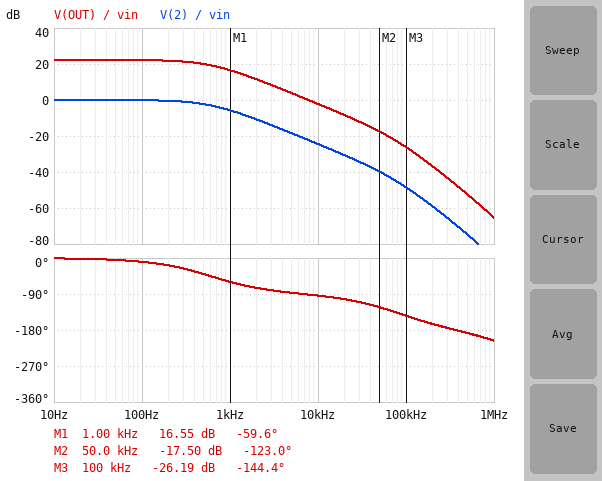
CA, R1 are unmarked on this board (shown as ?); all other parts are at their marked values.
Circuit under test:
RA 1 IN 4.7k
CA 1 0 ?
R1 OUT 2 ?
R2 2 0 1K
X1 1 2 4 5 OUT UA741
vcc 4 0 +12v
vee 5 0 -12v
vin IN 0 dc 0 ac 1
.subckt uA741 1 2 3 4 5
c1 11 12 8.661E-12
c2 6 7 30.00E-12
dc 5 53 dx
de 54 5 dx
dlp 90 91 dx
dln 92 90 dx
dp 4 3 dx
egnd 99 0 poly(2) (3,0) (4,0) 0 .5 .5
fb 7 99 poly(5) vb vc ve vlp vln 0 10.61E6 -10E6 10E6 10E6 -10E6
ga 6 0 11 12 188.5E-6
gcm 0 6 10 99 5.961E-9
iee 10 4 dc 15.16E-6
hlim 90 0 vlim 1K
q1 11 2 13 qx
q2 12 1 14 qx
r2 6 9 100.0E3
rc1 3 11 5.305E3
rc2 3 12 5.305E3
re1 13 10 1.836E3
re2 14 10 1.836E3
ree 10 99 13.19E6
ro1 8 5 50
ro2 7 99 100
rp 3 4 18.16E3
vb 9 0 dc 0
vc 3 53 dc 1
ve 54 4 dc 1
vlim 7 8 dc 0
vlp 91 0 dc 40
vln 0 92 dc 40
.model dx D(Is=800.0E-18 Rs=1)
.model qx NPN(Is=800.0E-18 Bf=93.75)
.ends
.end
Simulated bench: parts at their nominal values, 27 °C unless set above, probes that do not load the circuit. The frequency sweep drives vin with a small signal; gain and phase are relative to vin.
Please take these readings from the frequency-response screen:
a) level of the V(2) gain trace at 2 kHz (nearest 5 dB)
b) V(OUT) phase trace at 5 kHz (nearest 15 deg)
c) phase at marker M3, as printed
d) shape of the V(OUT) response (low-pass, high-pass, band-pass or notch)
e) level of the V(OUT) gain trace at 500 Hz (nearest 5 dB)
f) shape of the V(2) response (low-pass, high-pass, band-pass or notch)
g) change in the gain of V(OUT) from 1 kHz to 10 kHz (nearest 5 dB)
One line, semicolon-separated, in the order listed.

-10 dB; -90 deg; -144.4 deg; low-pass; 20 dB; low-pass; -20 dB
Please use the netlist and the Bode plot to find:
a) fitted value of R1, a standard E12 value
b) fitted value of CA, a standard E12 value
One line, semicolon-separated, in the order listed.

12 kΩ; 56 nF
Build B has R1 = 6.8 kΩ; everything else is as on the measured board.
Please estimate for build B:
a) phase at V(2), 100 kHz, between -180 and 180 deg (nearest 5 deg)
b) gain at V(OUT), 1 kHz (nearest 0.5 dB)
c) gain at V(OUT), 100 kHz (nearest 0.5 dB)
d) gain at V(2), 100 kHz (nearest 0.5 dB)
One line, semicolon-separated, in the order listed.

-130 deg; 12.0 dB; -28.5 dB; -46.0 dB
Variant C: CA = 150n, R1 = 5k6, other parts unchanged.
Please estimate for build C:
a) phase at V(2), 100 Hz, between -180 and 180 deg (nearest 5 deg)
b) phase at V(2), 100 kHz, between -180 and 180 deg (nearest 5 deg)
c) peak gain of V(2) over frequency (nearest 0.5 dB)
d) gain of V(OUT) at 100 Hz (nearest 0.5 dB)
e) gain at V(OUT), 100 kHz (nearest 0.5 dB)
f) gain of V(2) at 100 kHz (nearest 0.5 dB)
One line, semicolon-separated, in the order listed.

-25 deg; -125 deg; 0 dB; 15.5 dB; -38.0 dB; -54.5 dB
